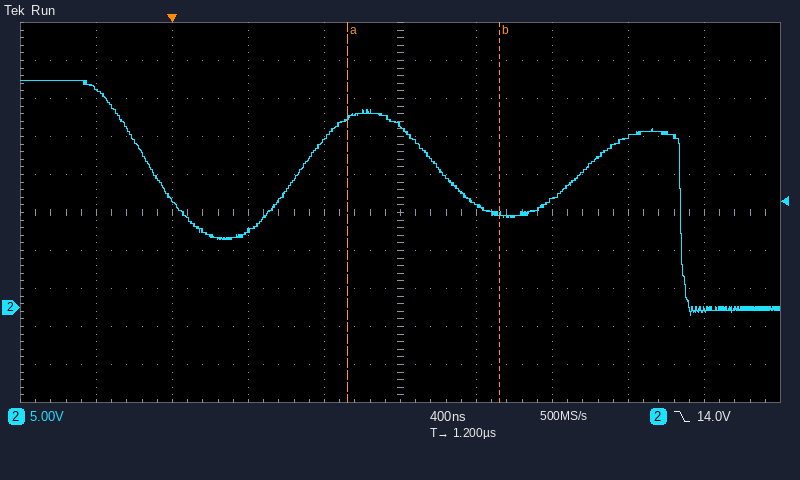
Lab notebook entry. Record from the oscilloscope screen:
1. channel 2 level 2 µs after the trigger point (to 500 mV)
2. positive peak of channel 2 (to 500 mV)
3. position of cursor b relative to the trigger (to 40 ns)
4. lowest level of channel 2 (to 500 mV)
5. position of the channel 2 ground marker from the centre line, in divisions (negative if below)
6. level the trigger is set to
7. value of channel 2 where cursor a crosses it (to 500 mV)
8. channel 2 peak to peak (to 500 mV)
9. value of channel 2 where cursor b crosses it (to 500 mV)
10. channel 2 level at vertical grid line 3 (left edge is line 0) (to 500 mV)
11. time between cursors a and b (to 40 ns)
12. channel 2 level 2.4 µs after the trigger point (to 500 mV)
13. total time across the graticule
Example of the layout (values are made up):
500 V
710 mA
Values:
14.0 V
30.0 V
+1.72 µs
-1.0 V
-2.5 div
14.0 V
25.0 V
31.0 V
12.5 V
10.0 V
800 ns
22.5 V
4 µs
